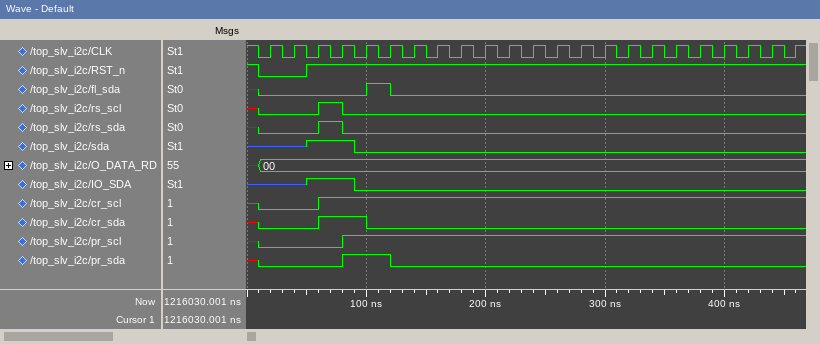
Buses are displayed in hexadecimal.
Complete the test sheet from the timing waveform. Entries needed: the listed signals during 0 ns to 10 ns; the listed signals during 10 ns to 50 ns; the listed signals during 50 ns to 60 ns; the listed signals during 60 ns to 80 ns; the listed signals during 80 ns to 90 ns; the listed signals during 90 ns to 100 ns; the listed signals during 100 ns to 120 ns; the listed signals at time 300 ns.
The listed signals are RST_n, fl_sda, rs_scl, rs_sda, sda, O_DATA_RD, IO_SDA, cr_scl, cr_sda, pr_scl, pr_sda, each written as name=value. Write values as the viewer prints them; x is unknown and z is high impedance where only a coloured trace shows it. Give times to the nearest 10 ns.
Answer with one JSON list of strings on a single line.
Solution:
["RST_n=1, fl_sda=x, rs_scl=x, rs_sda=x, sda=z, O_DATA_RD=x, IO_SDA=z, cr_scl=z, cr_sda=x, pr_scl=x, pr_sda=x", "RST_n=0, fl_sda=0, rs_scl=0, rs_sda=0, sda=z, O_DATA_RD=00, IO_SDA=z, cr_scl=0, cr_sda=0, pr_scl=0, pr_sda=0", "RST_n=1, fl_sda=0, rs_scl=0, rs_sda=0, sda=1, O_DATA_RD=00, IO_SDA=1, cr_scl=0, cr_sda=0, pr_scl=0, pr_sda=0", "RST_n=1, fl_sda=0, rs_scl=1, rs_sda=1, sda=1, O_DATA_RD=00, IO_SDA=1, cr_scl=1, cr_sda=1, pr_scl=0, pr_sda=0", "RST_n=1, fl_sda=0, rs_scl=0, rs_sda=0, sda=1, O_DATA_RD=00, IO_SDA=1, cr_scl=1, cr_sda=1, pr_scl=1, pr_sda=1", "RST_n=1, fl_sda=0, rs_scl=0, rs_sda=0, sda=0, O_DATA_RD=00, IO_SDA=0, cr_scl=1, cr_sda=1, pr_scl=1, pr_sda=1", "RST_n=1, fl_sda=1, rs_scl=0, rs_sda=0, sda=0, O_DATA_RD=00, IO_SDA=0, cr_scl=1, cr_sda=0, pr_scl=1, pr_sda=1", "RST_n=1, fl_sda=0, rs_scl=0, rs_sda=0, sda=0, O_DATA_RD=00, IO_SDA=0, cr_scl=1, cr_sda=0, pr_scl=1, pr_sda=0"]
